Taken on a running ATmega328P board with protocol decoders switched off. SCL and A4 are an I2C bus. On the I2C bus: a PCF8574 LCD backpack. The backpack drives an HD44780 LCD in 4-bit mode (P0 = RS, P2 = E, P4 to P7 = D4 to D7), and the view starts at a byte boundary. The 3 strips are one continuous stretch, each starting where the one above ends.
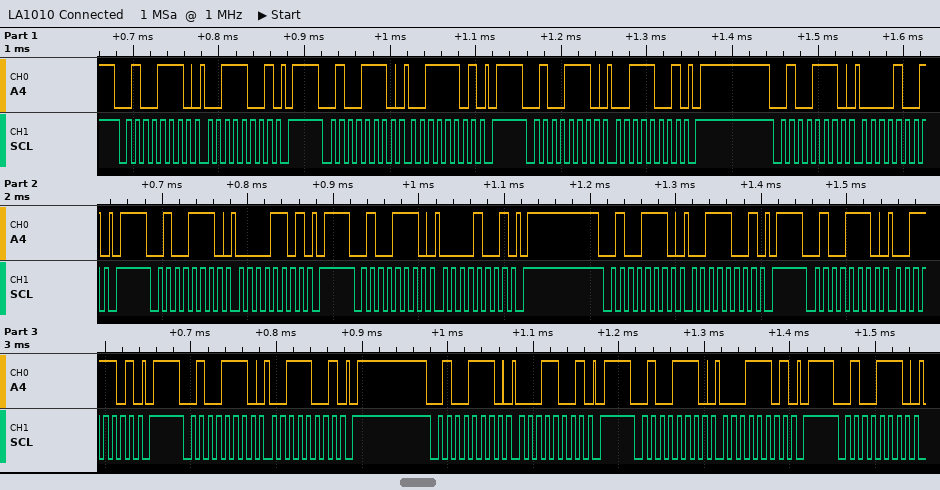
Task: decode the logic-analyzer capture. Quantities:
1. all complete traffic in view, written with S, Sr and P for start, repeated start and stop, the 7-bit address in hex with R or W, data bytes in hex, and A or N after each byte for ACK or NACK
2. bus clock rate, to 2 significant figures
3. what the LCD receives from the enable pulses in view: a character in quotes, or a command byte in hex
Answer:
S 27W A 39 A P S 27W A 3D A P S 27W A 39 A P S 27W A 09 A P S 27W A 0D A P S 27W A 09 A P S 27W A 39 A P S 27W A 3D A P S 27W A 39 A P S 27W A 19 A P S 27W A 1D A P S 27W A
100 kHz
'0'
